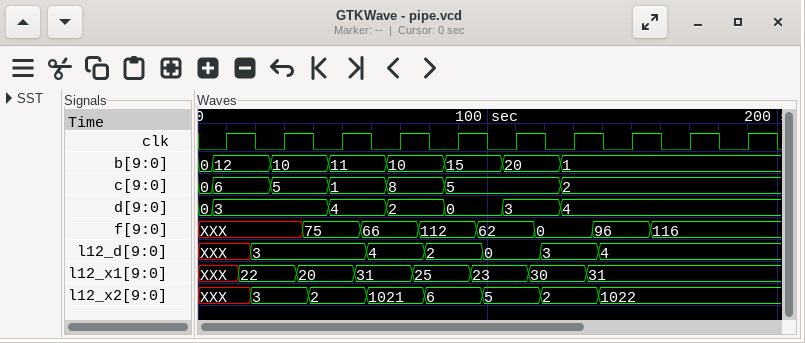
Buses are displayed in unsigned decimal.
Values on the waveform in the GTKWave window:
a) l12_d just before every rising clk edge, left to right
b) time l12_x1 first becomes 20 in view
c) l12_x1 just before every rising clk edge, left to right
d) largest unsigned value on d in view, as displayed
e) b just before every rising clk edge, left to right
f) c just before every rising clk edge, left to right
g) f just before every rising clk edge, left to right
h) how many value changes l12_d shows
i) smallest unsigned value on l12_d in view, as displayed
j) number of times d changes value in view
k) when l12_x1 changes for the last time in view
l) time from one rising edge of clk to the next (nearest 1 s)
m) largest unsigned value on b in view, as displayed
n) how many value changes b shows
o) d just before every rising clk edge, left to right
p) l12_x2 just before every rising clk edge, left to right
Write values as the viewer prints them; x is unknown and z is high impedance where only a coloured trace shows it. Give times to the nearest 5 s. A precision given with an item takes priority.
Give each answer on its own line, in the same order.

XXX, 3, 3, 4, 2, 0, 3, 4, 4, 4
35 s
XXX, 22, 20, 31, 25, 23, 30, 31, 31, 31
4
12, 10, 11, 10, 15, 20, 1, 1, 1, 1
6, 5, 1, 8, 5, 5, 2, 2, 2, 2
XXX, XXX, 75, 66, 112, 62, 0, 96, 116, 116
6
0
6
135 s
20 s
20
7
3, 3, 4, 2, 0, 3, 4, 4, 4, 4
XXX, 3, 2, 1021, 6, 5, 2, 1022, 1022, 1022
